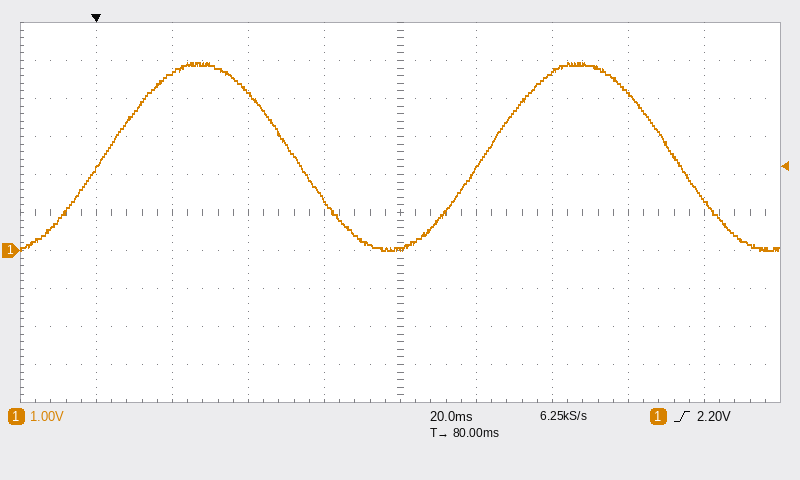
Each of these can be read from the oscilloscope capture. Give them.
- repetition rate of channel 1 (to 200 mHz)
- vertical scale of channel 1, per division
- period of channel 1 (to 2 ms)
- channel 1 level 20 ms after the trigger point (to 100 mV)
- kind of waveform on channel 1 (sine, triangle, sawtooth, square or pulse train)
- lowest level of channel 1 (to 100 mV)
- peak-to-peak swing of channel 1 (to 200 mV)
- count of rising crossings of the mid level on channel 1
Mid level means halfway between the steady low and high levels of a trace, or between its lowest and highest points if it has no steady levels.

10.0 Hz
1 V
100 ms
4.7 V
sine
0.0 V
5.0 V
2
